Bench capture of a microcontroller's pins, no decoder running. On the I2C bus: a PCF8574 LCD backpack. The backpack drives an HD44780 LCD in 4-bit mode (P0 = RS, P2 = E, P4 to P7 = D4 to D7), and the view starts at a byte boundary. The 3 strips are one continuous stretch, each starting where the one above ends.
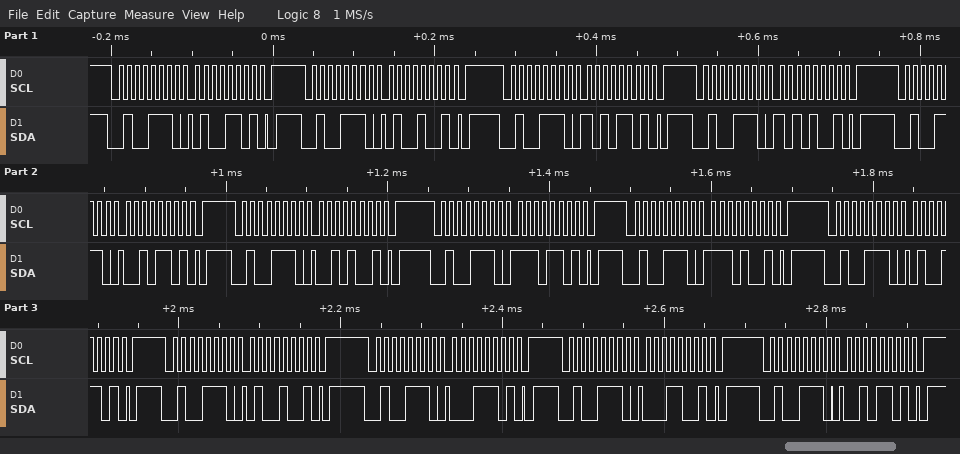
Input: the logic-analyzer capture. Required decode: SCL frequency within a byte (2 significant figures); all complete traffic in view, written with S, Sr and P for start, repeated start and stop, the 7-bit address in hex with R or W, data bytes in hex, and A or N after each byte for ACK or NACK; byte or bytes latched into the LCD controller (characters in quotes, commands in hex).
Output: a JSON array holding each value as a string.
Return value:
["100 kHz", "S 27W A 4D A P S 27W A 49 A P S 27W A AD A P S 27W A A9 A P S 27W A 2D A P S 27W A 29 A P S 27W A ED A P S 27W A E9 A P S 27W A 4D A P S 27W A 49 A P S 27W A 1D A P S 27W A 19 A P S 27W A 2D A P", "'J' '.' 'A'"]
